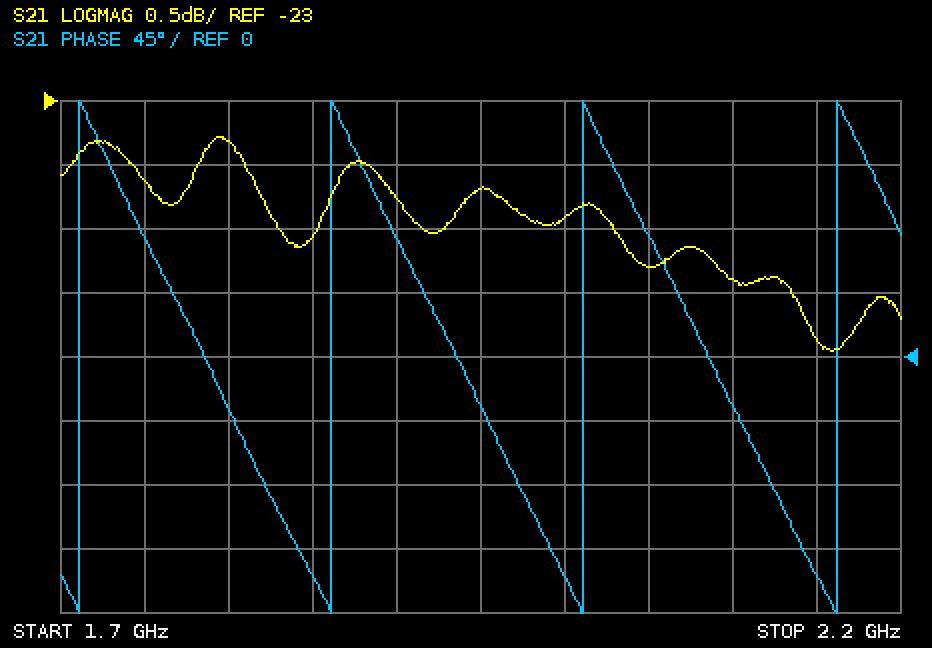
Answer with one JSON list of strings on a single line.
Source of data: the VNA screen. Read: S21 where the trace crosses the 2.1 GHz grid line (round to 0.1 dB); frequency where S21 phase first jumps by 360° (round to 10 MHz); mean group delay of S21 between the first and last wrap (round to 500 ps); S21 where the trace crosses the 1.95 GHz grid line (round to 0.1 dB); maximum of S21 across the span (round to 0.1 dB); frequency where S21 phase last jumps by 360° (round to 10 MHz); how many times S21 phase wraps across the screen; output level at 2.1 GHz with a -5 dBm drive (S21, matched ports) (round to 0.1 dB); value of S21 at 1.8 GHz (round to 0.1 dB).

["-24.4 dB", "1.71 GHz", "6.5 ns", "-23.7 dB", "-23.3 dB", "2.16 GHz", "4", "-29.4 dBm", "-23.3 dB"]
